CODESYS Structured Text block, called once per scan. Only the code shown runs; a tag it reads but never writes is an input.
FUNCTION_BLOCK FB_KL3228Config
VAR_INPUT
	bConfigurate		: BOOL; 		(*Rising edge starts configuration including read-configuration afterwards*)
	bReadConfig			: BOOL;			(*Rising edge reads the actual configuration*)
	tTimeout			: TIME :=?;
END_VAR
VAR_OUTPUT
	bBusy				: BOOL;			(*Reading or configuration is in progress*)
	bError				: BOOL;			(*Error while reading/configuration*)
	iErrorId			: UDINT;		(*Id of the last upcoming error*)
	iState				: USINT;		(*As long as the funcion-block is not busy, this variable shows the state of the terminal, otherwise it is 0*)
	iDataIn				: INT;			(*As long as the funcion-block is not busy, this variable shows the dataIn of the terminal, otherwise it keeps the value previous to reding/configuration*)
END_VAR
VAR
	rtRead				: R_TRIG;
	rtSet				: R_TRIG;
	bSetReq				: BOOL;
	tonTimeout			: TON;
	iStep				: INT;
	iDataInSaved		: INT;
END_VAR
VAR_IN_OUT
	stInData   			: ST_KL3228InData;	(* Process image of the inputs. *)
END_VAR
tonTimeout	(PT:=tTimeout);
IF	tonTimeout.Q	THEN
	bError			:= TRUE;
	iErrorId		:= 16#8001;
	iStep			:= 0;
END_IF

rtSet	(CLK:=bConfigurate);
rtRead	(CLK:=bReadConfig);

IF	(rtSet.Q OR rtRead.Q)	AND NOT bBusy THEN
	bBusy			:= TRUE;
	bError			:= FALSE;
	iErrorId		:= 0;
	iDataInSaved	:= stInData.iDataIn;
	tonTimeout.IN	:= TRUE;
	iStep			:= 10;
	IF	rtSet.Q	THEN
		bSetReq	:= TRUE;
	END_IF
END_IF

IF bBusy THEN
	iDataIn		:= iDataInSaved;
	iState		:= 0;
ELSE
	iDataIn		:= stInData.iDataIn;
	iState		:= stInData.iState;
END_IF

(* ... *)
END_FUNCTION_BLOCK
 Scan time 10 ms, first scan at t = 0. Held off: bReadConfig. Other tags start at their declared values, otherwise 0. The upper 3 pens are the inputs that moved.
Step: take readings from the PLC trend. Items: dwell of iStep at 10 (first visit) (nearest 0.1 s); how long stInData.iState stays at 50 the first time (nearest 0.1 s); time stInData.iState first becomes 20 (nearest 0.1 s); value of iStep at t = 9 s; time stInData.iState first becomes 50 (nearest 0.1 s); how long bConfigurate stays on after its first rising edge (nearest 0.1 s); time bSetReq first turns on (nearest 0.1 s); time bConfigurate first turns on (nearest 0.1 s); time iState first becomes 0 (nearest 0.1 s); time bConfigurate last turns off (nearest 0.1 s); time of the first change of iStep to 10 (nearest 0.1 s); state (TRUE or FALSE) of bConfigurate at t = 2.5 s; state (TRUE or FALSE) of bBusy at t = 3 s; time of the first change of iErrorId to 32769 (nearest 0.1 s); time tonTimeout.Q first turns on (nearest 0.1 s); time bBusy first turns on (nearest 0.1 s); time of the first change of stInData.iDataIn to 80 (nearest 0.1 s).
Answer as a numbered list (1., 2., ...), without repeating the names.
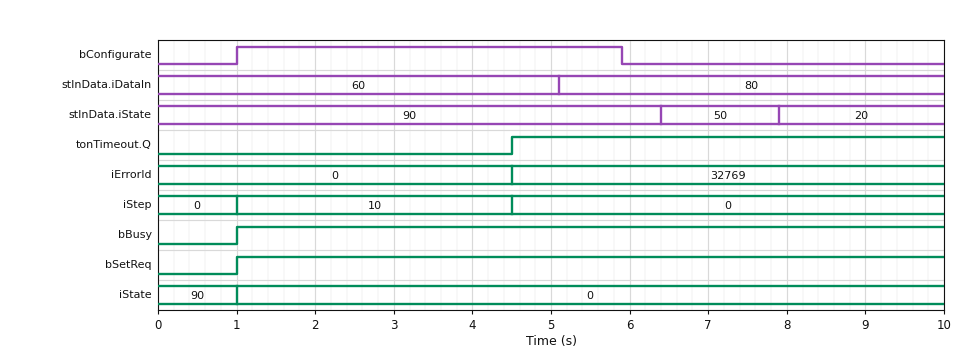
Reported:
1. 3.5 s
2. 1.5 s
3. 7.9 s
4. 0
5. 6.4 s
6. 4.9 s
7. 1.0 s
8. 1.0 s
9. 1.0 s
10. 5.9 s
11. 1.0 s
12. TRUE
13. TRUE
14. 4.5 s
15. 4.5 s
16. 1.0 s
17. 5.1 s
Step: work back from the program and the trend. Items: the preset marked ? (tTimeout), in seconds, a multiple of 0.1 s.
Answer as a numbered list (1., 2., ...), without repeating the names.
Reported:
1. 3.5 s
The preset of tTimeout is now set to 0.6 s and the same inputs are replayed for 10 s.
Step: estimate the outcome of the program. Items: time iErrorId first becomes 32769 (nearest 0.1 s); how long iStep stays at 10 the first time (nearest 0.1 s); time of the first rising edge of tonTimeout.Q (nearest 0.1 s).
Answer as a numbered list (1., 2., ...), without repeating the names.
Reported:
1. 1.6 s
2. 0.6 s
3. 1.6 s
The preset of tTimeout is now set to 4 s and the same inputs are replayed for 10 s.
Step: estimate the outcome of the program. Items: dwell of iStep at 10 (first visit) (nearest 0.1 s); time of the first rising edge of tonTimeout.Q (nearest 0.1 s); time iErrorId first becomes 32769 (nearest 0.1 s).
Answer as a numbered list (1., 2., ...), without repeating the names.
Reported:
1. 4.0 s
2. 5.0 s
3. 5.0 s
